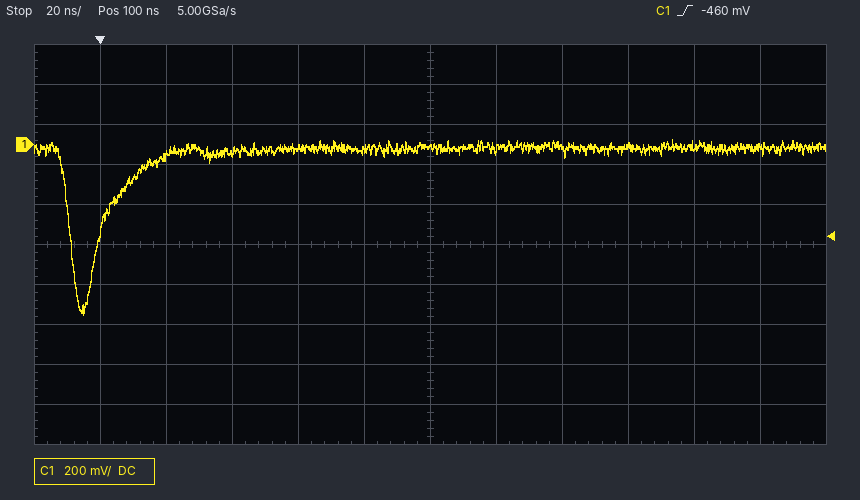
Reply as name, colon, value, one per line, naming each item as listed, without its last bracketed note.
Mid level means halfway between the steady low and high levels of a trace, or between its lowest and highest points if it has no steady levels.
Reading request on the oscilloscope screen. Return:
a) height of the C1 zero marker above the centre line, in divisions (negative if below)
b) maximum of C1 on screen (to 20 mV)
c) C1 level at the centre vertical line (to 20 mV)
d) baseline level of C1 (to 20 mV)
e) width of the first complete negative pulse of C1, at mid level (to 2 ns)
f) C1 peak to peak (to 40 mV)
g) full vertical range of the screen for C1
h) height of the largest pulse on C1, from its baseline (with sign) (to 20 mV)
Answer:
height of the C1 zero marker above the centre line, in divisions: +2.5 div
maximum of C1 on screen: 20 mV
C1 level at the centre vertical line: -20 mV
baseline level of C1: -20 mV
width of the first complete negative pulse of C1, at mid level: 10 ns
C1 peak to peak: 880 mV
full vertical range of the screen for C1: 2 V
height of the largest pulse on C1, from its baseline (with sign): -840 mV
